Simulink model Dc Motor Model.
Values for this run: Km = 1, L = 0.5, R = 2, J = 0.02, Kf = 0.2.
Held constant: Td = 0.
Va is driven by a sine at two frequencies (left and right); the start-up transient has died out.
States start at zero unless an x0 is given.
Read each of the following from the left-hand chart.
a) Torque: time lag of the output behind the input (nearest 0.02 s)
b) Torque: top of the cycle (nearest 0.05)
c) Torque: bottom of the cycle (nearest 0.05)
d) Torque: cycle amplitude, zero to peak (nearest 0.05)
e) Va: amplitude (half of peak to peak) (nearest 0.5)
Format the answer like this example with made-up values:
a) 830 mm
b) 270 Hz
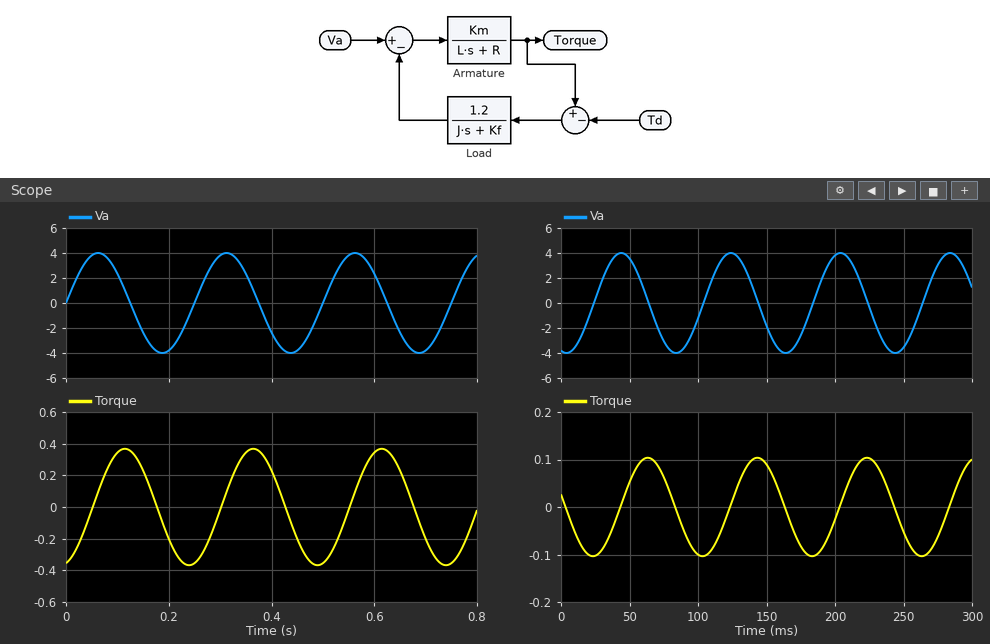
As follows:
a) 0.06 s
b) 0.35
c) -0.35
d) 0.35
e) 4.0
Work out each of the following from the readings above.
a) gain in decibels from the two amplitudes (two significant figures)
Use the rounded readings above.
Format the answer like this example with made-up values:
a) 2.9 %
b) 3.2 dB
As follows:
a) -21 dB
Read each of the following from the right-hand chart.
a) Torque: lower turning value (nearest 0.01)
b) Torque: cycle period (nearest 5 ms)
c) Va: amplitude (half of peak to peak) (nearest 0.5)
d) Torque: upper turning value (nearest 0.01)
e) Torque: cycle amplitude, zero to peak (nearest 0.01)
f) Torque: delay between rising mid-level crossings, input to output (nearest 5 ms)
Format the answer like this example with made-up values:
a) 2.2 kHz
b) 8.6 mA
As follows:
a) -0.10
b) 80 ms
c) 4.0
d) 0.10
e) 0.10
f) 20 ms
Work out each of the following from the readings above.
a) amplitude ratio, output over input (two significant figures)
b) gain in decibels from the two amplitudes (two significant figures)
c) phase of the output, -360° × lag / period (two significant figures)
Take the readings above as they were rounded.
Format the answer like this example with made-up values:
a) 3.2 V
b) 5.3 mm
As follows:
a) 0.025
b) -32 dB
c) -90°
